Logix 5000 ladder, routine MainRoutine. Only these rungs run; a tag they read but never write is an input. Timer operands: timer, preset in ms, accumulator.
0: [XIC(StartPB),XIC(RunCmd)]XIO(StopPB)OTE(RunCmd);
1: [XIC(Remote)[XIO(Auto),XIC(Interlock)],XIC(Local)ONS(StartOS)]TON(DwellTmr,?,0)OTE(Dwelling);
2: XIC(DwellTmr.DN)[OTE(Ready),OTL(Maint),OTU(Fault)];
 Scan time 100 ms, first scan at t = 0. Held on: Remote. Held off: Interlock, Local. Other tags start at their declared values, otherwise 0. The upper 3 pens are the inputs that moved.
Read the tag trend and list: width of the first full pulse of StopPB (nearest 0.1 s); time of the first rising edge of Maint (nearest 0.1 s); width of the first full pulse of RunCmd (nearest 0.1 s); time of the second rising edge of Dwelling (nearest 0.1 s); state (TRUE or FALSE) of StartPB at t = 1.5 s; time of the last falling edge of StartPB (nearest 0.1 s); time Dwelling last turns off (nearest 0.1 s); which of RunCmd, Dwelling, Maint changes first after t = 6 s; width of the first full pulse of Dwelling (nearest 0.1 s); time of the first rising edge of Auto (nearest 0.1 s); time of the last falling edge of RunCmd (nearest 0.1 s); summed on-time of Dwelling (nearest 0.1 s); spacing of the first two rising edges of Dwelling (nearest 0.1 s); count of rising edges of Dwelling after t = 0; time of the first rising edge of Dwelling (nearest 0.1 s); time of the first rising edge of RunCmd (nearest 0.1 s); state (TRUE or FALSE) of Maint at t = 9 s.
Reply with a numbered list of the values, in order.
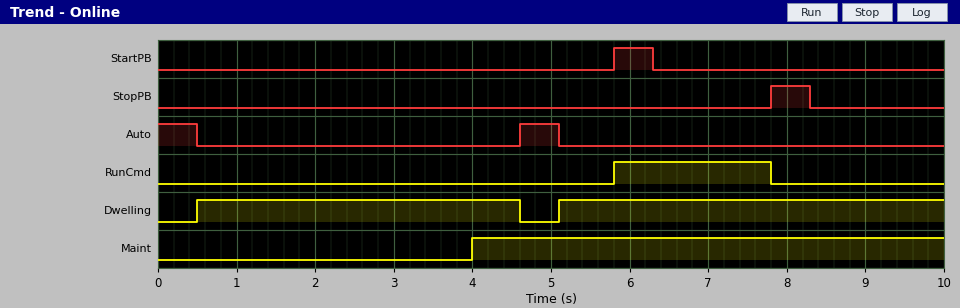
1. 0.5 s
2. 4.0 s
3. 2.0 s
4. 5.1 s
5. FALSE
6. 6.3 s
7. 4.6 s
8. RunCmd
9. 4.1 s
10. 4.6 s
11. 7.8 s
12. 9.0 s
13. 4.6 s
14. 2
15. 0.5 s
16. 5.8 s
17. TRUE
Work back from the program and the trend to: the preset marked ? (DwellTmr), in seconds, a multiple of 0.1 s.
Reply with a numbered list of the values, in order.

1. 3.5 s
